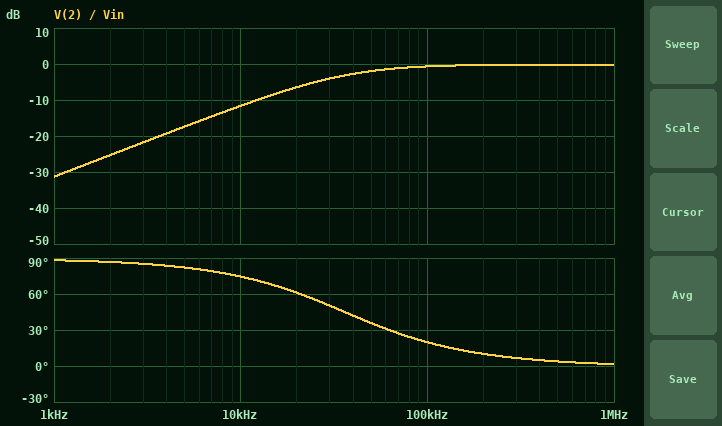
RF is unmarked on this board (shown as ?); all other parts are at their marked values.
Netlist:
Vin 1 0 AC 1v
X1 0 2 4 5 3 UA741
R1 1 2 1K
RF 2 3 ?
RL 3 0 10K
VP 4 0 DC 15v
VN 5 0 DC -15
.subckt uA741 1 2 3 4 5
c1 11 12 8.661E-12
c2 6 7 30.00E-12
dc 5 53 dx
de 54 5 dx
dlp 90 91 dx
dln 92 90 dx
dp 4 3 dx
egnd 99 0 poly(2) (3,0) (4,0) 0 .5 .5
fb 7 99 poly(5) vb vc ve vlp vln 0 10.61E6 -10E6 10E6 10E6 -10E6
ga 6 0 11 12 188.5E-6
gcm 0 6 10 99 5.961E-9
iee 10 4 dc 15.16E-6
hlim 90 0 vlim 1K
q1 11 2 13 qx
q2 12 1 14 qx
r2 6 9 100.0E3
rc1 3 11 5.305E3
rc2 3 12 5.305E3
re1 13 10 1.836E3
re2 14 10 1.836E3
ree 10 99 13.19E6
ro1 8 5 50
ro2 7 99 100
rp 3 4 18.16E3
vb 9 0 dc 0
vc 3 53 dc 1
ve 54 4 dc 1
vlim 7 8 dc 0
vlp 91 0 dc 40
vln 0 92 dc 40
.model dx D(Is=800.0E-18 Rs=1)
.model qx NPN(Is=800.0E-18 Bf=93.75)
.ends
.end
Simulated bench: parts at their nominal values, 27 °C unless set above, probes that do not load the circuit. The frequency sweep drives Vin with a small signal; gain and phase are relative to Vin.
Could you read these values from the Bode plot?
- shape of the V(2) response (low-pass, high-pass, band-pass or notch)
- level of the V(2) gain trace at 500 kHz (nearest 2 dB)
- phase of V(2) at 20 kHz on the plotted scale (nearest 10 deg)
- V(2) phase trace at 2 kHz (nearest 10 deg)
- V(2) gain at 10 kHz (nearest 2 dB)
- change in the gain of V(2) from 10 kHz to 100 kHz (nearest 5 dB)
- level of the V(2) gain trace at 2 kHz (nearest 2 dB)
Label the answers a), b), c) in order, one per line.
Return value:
a) high-pass
b) 0 dB
c) 60 deg
d) 90 deg
e) -12 dB
f) 10 dB
g) -26 dB
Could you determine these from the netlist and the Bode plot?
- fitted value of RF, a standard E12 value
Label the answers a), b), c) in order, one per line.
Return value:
a) 27 kΩ
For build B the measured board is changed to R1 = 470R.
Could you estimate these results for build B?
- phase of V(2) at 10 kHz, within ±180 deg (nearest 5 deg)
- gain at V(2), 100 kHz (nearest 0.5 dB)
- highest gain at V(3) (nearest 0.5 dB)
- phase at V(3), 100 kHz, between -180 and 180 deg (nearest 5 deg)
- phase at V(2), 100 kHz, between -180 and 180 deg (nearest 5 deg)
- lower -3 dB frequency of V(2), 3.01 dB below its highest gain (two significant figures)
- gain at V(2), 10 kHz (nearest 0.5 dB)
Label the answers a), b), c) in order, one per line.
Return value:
a) 60 deg
b) 0 dB
c) 35.0 dB
d) 95 deg
e) 10 deg
f) 17 kHz
g) -6.0 dB
